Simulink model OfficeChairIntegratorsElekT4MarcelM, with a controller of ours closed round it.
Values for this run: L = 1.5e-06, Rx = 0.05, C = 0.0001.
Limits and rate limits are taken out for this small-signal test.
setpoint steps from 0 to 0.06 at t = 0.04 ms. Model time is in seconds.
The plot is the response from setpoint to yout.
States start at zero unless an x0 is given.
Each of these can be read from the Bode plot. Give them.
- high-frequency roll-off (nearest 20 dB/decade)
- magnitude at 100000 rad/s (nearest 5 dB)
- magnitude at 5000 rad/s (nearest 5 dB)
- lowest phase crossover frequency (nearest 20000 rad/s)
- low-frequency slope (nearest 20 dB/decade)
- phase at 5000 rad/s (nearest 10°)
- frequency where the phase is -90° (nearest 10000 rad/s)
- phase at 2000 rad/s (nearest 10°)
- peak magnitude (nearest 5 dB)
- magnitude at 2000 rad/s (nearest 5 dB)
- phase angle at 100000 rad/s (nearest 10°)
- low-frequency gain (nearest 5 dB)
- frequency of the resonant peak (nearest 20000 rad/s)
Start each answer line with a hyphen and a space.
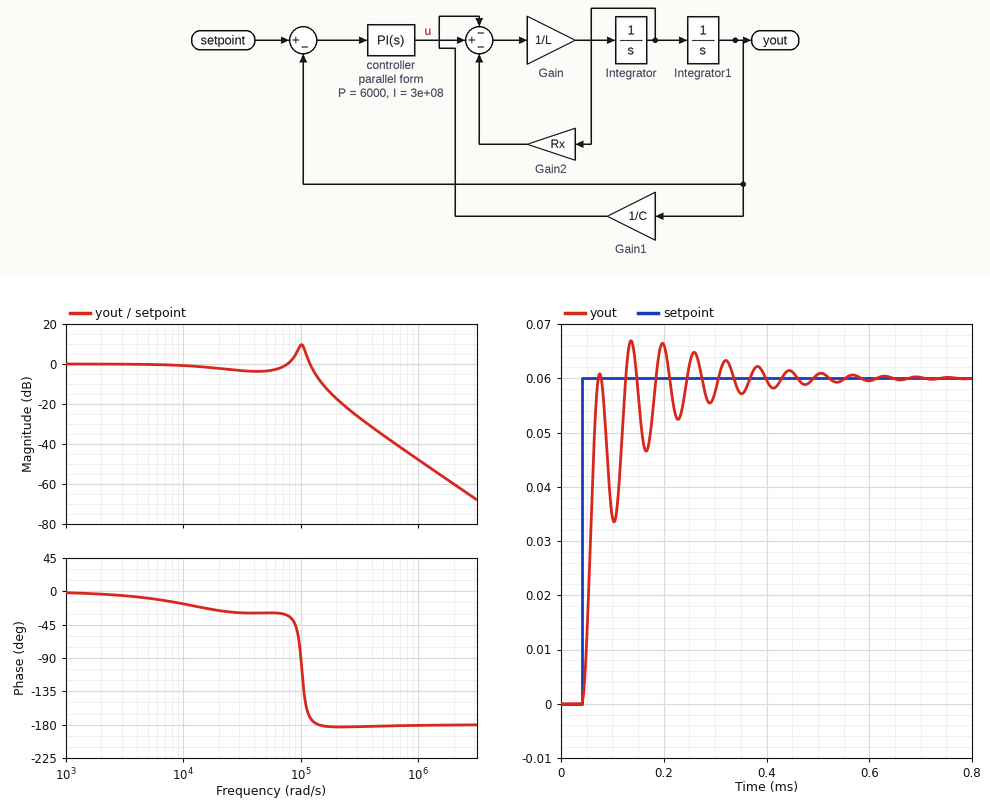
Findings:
- -40 dB/decade
- 10 dB
- 0 dB
- 140000 rad/s
- 0 dB/decade
- -10°
- 100000 rad/s
- 0°
- 10 dB
- 0 dB
- -90°
- 0 dB
- 100000 rad/s
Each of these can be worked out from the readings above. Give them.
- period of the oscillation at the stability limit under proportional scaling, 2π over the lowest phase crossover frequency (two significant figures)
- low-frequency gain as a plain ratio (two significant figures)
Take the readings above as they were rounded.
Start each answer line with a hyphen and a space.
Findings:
- 0.000045 s
- 1.0
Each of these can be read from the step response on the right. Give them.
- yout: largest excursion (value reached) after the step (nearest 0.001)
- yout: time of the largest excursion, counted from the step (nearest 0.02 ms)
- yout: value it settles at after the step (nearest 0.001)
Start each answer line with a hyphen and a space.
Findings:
- 0.067
- 0.10 ms
- 0.060
